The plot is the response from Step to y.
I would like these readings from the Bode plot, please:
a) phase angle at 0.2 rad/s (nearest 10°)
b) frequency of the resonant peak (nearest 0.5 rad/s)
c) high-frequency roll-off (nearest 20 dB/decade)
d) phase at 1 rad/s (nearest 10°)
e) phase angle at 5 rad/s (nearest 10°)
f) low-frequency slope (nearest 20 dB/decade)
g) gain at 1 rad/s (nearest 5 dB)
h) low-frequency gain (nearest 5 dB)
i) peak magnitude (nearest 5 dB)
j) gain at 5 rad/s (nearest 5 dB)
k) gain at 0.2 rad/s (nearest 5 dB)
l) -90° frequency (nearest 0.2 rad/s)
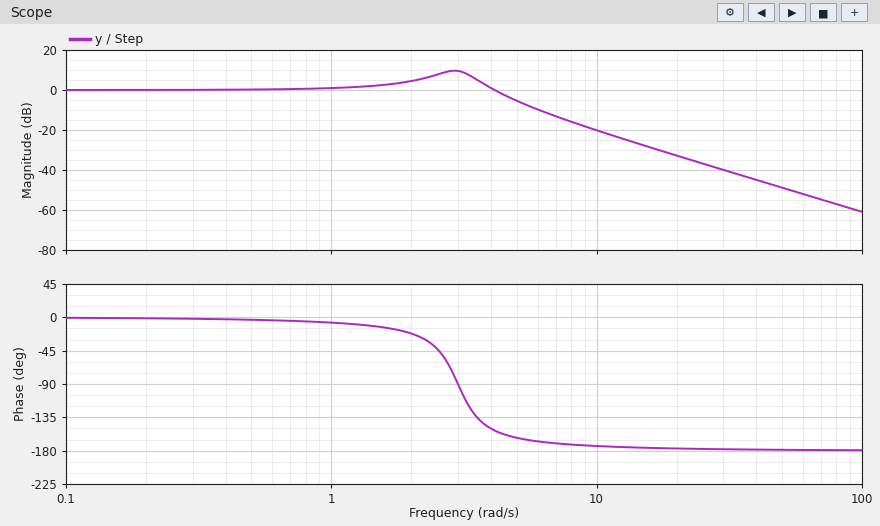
0°
3.0 rad/s
-40 dB/decade
-10°
-160°
0 dB/decade
0 dB
0 dB
10 dB
-5 dB
0 dB
3.0 rad/s
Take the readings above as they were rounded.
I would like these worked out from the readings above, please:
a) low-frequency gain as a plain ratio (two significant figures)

1.0
